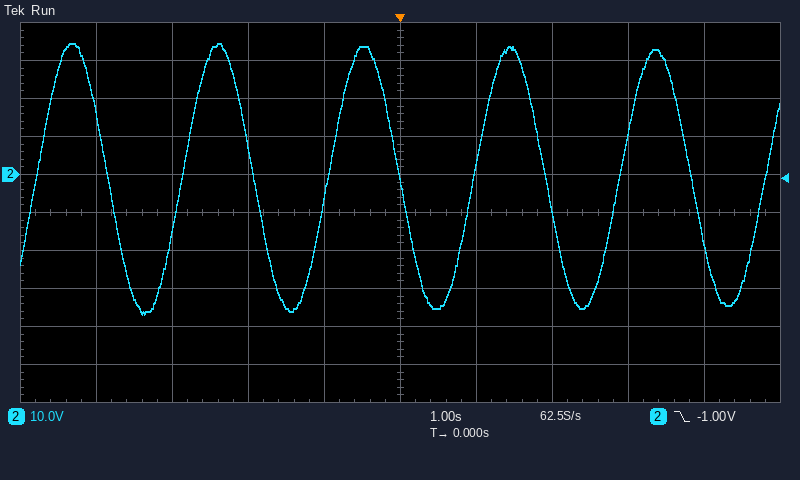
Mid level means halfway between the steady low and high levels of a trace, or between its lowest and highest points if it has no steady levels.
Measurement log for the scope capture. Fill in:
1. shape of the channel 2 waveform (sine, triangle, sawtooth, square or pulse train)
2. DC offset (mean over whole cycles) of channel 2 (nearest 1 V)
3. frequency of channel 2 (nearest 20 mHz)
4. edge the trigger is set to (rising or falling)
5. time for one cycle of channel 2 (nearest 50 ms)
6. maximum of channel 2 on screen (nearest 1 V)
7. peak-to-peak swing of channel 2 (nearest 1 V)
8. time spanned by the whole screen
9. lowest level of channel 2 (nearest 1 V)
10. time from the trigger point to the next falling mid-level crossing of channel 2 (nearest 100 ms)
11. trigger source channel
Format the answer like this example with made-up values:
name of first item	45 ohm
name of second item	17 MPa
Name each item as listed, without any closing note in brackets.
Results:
shape of the channel 2 waveform	sine
DC offset (mean over whole cycles) of channel 2	-1 V
frequency of channel 2	520 mHz
edge the trigger is set to	falling
time for one cycle of channel 2	1.90 s
maximum of channel 2 on screen	34 V
peak-to-peak swing of channel 2	71 V
time spanned by the whole screen	10 s
lowest level of channel 2	-37 V
time from the trigger point to the next falling mid-level crossing of channel 2	1.9 s
trigger source channel	channel 2
